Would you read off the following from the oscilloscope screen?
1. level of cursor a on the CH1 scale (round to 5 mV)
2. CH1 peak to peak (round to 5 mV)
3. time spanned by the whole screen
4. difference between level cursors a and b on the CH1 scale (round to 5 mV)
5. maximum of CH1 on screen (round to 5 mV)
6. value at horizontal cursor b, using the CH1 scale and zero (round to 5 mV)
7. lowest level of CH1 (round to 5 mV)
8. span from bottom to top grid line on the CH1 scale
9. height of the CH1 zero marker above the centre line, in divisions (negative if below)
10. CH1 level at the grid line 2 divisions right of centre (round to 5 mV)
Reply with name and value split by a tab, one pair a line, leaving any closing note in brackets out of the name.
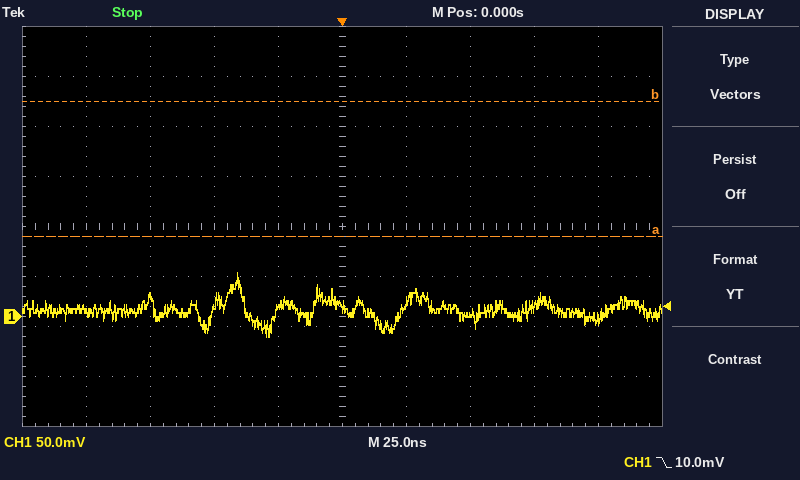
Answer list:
level of cursor a on the CH1 scale	80 mV
CH1 peak to peak	65 mV
time spanned by the whole screen	250 ns
difference between level cursors a and b on the CH1 scale	135 mV
maximum of CH1 on screen	45 mV
value at horizontal cursor b, using the CH1 scale and zero	215 mV
lowest level of CH1	-20 mV
span from bottom to top grid line on the CH1 scale	400 mV
height of the CH1 zero marker above the centre line, in divisions	-1.8 div
CH1 level at the grid line 2 divisions right of centre	5 mV
